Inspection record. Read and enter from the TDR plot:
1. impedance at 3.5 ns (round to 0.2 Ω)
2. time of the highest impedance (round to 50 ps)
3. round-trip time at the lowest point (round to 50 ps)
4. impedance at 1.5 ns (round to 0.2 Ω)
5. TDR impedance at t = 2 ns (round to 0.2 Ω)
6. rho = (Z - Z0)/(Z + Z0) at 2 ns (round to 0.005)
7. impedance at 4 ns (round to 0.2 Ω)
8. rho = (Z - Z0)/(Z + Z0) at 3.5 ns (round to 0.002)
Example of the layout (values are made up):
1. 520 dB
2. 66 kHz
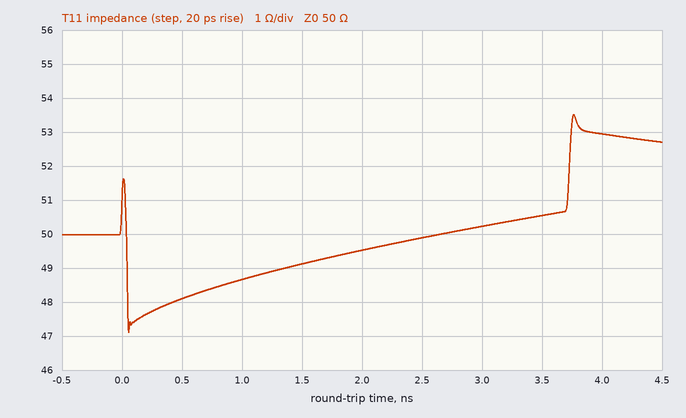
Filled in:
1. 50.6 Ω
2. 3.75 ns
3. 50 ps
4. 49.2 Ω
5. 49.6 Ω
6. -0.005
7. 53.0 Ω
8. +0.006
